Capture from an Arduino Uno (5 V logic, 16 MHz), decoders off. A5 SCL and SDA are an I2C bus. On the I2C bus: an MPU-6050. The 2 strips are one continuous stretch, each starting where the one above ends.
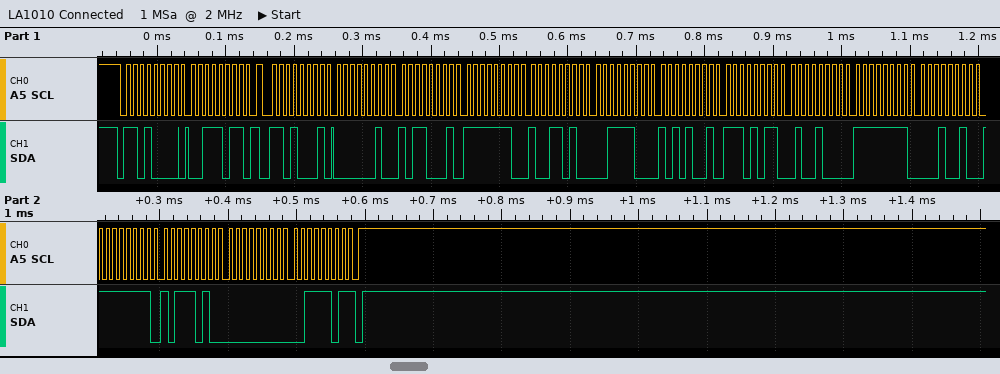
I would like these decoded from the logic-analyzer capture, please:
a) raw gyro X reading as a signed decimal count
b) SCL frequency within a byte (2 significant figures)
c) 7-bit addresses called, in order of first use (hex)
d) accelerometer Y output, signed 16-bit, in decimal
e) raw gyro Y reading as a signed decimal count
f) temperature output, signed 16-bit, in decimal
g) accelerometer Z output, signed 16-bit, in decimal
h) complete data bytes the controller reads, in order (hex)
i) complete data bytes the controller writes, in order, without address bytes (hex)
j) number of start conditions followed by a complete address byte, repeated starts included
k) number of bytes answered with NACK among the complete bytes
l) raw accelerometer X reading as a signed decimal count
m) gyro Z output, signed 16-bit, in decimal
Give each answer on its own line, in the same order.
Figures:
-238
100 kHz
0x68
-358
-70
-5304
15529
02 B1 FE 9A 3C A9 EB 48 FF 12 FF BA 00 3D
3B
2
1
689
61
